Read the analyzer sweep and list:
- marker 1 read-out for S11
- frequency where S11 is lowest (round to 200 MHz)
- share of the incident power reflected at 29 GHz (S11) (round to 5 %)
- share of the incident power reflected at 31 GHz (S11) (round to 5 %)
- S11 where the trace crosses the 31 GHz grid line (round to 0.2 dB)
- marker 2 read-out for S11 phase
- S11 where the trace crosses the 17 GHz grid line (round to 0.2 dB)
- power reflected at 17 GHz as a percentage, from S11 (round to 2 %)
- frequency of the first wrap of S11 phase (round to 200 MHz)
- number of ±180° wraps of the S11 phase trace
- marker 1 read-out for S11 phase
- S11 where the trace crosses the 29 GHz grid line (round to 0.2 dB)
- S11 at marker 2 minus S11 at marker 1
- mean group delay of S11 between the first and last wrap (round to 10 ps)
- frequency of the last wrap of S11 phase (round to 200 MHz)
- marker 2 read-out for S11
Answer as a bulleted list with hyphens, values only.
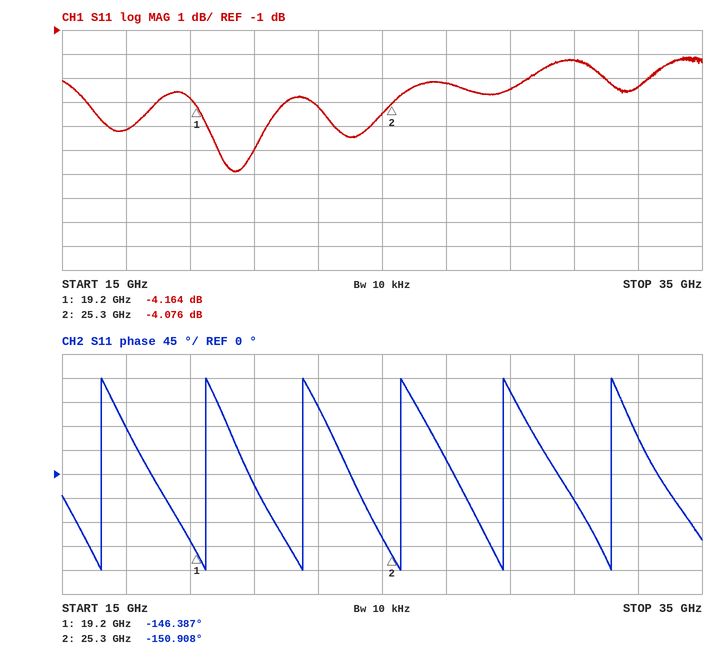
- -4.164 dB
- 20.4 GHz
- 45 %
- 60 %
- -2.2 dB
- -150.908°
- -5.2 dB
- 30 %
- 16.2 GHz
- 6
- -146.387°
- -3.4 dB
- 0.088 dB
- 310 ps
- 32.2 GHz
- -4.076 dB
